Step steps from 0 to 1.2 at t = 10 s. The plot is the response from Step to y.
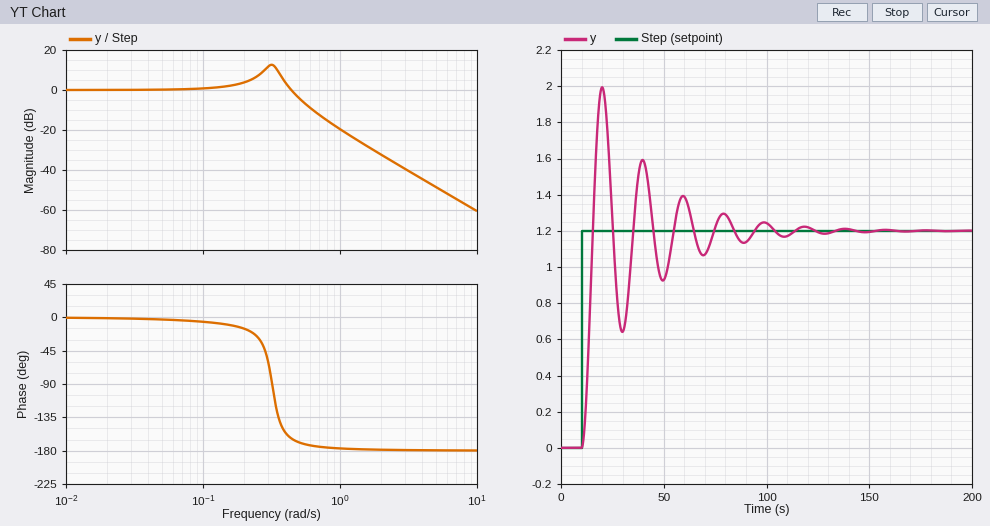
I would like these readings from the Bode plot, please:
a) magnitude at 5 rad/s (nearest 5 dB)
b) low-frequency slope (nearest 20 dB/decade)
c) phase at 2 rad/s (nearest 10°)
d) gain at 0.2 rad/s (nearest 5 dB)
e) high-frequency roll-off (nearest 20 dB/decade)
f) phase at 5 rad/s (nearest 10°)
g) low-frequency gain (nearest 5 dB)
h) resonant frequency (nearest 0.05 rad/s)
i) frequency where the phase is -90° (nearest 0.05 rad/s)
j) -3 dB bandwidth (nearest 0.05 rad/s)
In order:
-50 dB
0 dB/decade
-180°
5 dB
-40 dB/decade
-180°
0 dB
0.30 rad/s
0.30 rad/s
0.50 rad/s
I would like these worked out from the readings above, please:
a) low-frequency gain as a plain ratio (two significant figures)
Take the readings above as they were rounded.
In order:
1.0
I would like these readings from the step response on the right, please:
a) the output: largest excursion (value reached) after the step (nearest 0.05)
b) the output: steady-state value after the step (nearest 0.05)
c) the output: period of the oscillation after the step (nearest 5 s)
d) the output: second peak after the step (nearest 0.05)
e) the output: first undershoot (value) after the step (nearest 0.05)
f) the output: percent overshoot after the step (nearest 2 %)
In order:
2.00
1.20
20 s
1.60
0.65
66 %
